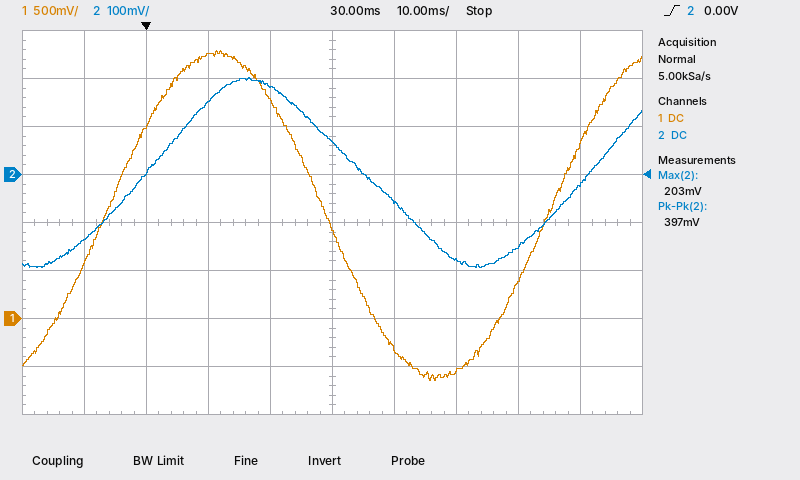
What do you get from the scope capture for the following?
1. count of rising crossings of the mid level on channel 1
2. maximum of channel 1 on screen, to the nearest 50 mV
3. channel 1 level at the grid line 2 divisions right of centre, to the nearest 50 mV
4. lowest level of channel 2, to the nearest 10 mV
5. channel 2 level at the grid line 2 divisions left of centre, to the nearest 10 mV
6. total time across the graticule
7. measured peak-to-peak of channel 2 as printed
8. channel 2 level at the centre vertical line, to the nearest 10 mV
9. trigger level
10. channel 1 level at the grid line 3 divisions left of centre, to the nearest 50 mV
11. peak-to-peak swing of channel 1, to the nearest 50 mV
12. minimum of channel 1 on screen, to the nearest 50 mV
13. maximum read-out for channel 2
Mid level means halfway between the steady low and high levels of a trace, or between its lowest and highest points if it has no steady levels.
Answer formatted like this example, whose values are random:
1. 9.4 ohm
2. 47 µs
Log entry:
1. 2
2. 2.80 V
3. -550 mV
4. -190 mV
5. 150 mV
6. 100 ms
7. 397 mV
8. 70 mV
9. 0.00 V
10. 2.00 V
11. 3.45 V
12. -650 mV
13. 203 mV
